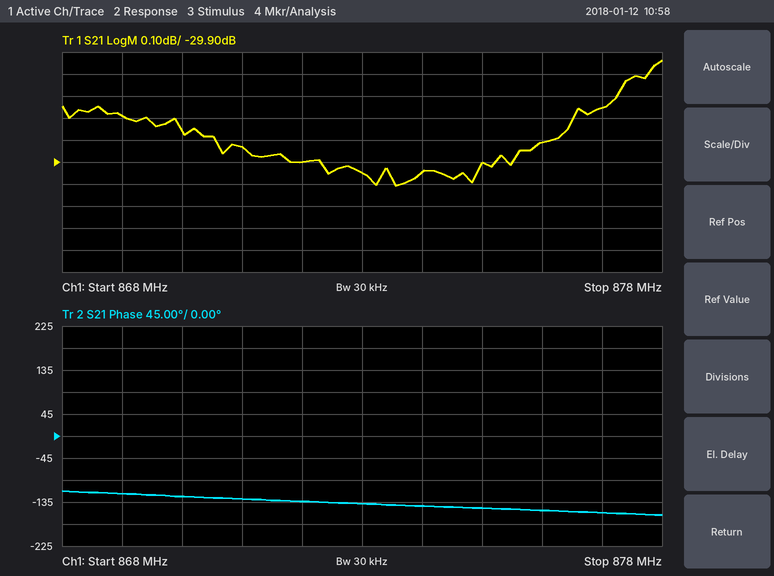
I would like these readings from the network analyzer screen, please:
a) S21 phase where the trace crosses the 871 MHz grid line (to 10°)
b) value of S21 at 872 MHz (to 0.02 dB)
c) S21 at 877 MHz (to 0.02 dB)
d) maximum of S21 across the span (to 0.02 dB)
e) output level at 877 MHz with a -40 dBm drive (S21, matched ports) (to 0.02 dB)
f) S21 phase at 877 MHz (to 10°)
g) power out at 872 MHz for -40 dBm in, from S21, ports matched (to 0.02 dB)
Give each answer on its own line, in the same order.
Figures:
-130°
-29.90 dB
-29.66 dB
-29.44 dB
-69.66 dBm
-160°
-69.90 dBm
